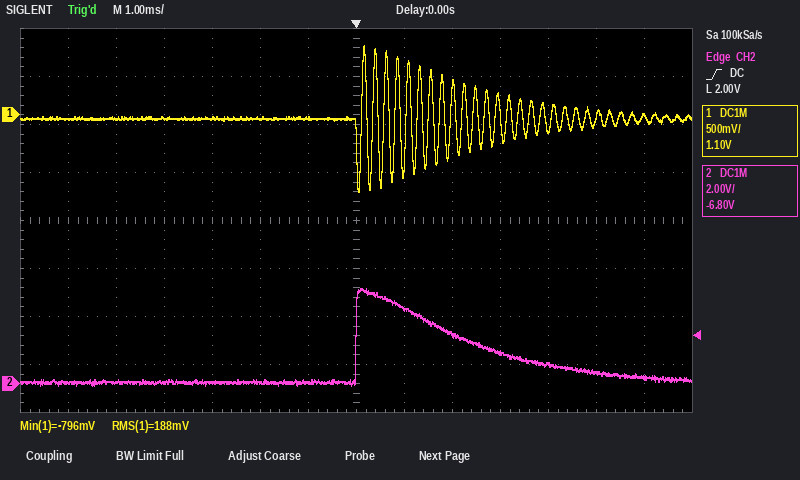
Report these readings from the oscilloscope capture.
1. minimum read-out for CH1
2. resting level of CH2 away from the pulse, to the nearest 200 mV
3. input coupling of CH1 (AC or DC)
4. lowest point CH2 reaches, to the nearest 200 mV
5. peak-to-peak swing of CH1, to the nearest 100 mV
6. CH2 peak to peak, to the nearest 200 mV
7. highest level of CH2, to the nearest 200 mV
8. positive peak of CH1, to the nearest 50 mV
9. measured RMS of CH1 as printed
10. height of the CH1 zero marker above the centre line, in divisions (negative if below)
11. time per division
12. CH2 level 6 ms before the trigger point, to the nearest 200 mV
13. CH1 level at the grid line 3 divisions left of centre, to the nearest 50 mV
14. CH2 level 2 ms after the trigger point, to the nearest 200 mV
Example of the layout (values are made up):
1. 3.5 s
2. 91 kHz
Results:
1. -796 mV
2. 0.0 V
3. DC
4. 0.0 V
5. 1.50 V
6. 4.0 V
7. 4.0 V
8. 700 mV
9. 188 mV
10. +2.2 div
11. 1 ms
12. 0.0 V
13. -50 mV
14. 2.0 V
